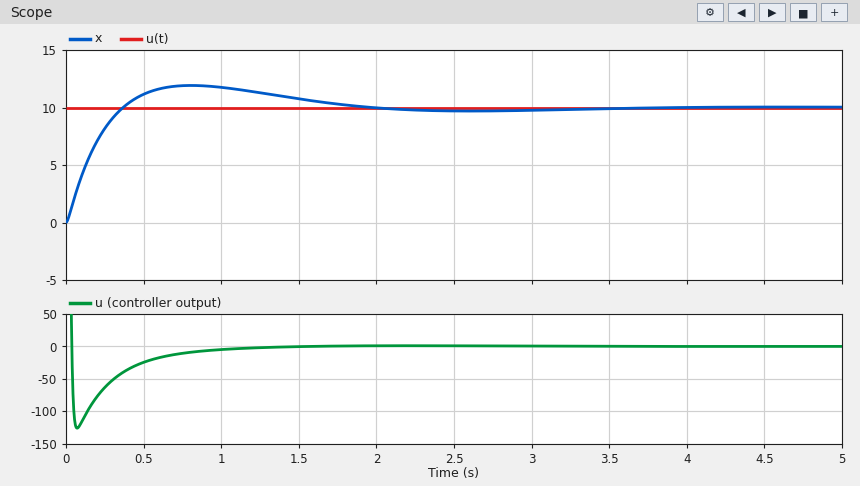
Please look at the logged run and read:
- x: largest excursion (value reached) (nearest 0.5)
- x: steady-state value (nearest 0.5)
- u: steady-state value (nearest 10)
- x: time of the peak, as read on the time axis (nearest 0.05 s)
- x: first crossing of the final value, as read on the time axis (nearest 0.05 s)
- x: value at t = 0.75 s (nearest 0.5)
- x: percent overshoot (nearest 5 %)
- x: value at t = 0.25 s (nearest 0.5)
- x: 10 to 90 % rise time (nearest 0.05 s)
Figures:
12.0
10.0
0
0.80 s
0.35 s
12.0
20 %
8.0
0.25 s
